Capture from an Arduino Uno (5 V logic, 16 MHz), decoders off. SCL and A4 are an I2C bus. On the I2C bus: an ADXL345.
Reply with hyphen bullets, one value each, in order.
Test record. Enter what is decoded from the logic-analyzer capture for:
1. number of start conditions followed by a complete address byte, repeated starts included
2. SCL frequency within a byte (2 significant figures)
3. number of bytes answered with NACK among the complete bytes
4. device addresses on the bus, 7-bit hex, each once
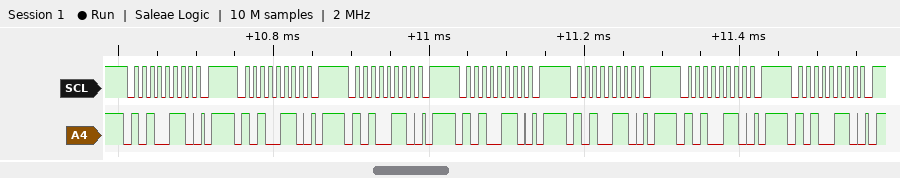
- 7
- 100 kHz
- 0
- 0x53
